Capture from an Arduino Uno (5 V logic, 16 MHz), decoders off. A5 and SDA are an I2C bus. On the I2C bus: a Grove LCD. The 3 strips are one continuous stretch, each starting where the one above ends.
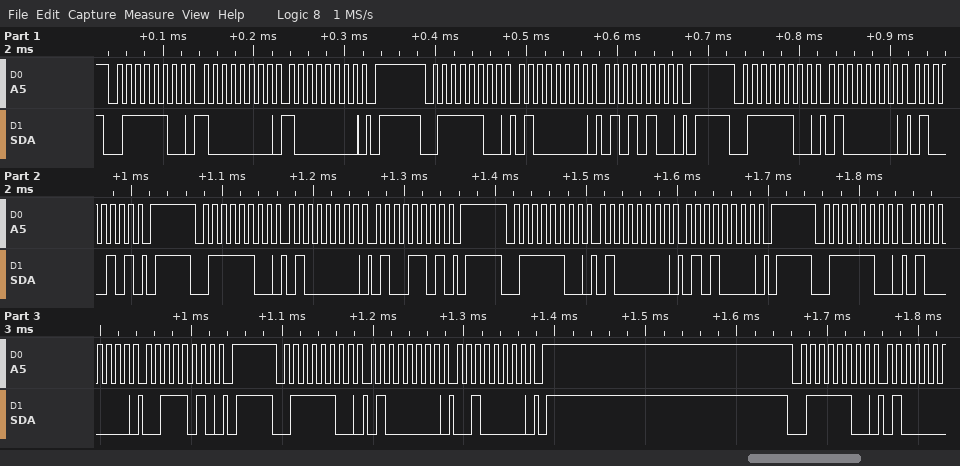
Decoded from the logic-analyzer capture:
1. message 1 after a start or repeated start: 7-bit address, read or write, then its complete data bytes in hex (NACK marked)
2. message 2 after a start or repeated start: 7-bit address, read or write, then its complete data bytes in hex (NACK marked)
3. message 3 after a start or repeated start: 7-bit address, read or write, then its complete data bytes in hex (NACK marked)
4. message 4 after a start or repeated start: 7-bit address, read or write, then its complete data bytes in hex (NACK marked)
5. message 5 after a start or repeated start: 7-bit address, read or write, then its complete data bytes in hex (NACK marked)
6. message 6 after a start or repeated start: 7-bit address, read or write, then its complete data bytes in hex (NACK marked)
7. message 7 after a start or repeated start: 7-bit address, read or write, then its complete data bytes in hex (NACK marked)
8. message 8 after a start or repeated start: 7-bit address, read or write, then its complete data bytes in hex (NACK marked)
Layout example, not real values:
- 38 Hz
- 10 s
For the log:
- 0x3E write: 80 80
- 0x3E write: 40 54
- 0x3E write: 40 45
- 0x3E write: 40 4D
- 0x3E write: 40 50
- 0x3E write: 40 3A
- 0x3E write: 40 20
- 0x3E write
